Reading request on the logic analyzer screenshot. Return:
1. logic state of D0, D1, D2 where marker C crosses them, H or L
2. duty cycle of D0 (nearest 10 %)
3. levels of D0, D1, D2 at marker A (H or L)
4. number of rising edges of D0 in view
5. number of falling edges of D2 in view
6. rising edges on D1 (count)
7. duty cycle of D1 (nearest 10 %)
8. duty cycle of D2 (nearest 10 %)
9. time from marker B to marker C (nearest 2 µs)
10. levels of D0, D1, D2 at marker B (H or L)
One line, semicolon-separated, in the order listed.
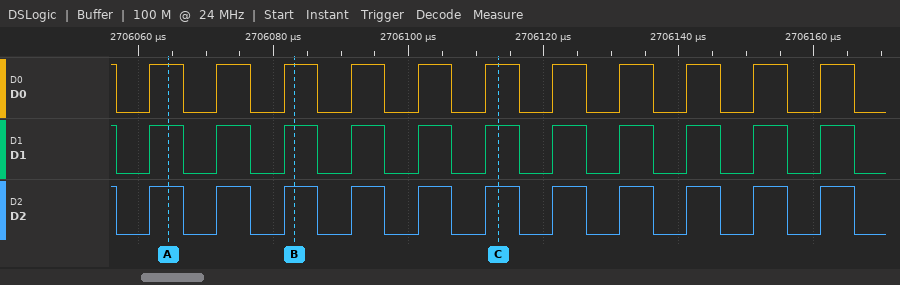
D0=H, D1=H, D2=H; 50 %; D0=H, D1=H, D2=H; 11; 12; 11; 50 %; 50 %; 30 µs; D0=H, D1=H, D2=H
